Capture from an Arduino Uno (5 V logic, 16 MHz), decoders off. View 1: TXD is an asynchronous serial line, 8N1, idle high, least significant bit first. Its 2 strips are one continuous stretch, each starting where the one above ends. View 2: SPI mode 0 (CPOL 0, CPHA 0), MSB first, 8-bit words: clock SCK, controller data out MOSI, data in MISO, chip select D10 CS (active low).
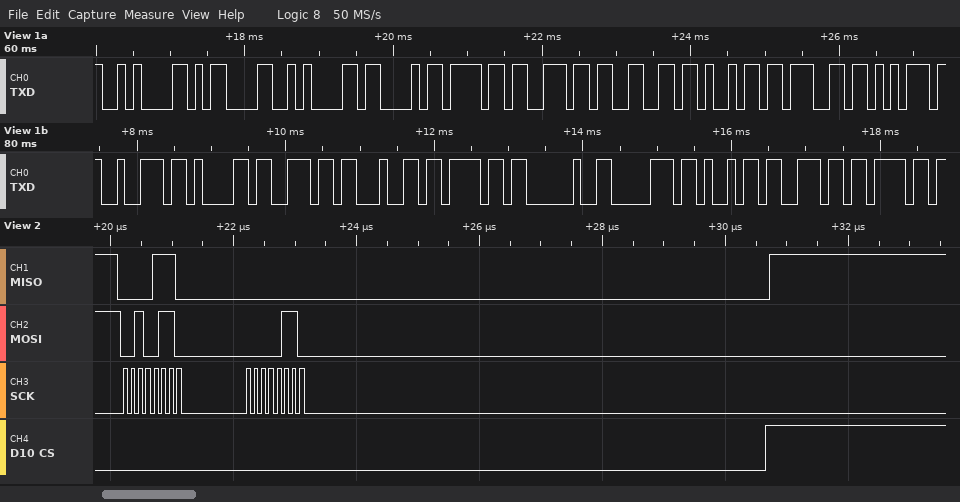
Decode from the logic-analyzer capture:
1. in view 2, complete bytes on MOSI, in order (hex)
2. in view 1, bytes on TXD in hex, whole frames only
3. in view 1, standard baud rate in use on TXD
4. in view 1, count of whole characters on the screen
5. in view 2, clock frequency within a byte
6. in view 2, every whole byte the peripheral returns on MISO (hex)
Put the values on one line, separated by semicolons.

26 06; 0x0A 0x0D 0x0A 0x43 0x6F 0x6E 0x66 0x69 0x67 0x75 0x72 0x61 0x6E 0x64 0x6F 0x20 0x70 0x69 0x6E 0x6F; 9600 baud; 20; 8 MHz; 0E 00
